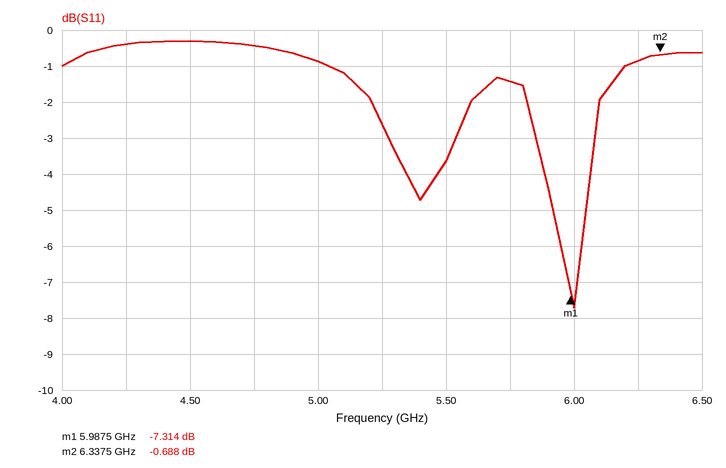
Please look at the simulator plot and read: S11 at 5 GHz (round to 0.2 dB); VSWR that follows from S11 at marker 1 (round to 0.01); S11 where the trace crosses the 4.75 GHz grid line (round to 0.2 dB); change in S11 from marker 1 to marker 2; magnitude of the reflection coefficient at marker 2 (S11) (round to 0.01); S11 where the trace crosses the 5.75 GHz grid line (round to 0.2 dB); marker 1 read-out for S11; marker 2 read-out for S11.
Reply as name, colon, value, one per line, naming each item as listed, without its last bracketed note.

S11 at 5 GHz: -0.8 dB
VSWR that follows from S11 at marker 1: 2.51
S11 where the trace crosses the 4.75 GHz grid line: -0.4 dB
change in S11 from marker 1 to marker 2: 6.626 dB
magnitude of the reflection coefficient at marker 2 (S11): 0.92
S11 where the trace crosses the 5.75 GHz grid line: -1.4 dB
marker 1 read-out for S11: -7.314 dB
marker 2 read-out for S11: -0.688 dB
